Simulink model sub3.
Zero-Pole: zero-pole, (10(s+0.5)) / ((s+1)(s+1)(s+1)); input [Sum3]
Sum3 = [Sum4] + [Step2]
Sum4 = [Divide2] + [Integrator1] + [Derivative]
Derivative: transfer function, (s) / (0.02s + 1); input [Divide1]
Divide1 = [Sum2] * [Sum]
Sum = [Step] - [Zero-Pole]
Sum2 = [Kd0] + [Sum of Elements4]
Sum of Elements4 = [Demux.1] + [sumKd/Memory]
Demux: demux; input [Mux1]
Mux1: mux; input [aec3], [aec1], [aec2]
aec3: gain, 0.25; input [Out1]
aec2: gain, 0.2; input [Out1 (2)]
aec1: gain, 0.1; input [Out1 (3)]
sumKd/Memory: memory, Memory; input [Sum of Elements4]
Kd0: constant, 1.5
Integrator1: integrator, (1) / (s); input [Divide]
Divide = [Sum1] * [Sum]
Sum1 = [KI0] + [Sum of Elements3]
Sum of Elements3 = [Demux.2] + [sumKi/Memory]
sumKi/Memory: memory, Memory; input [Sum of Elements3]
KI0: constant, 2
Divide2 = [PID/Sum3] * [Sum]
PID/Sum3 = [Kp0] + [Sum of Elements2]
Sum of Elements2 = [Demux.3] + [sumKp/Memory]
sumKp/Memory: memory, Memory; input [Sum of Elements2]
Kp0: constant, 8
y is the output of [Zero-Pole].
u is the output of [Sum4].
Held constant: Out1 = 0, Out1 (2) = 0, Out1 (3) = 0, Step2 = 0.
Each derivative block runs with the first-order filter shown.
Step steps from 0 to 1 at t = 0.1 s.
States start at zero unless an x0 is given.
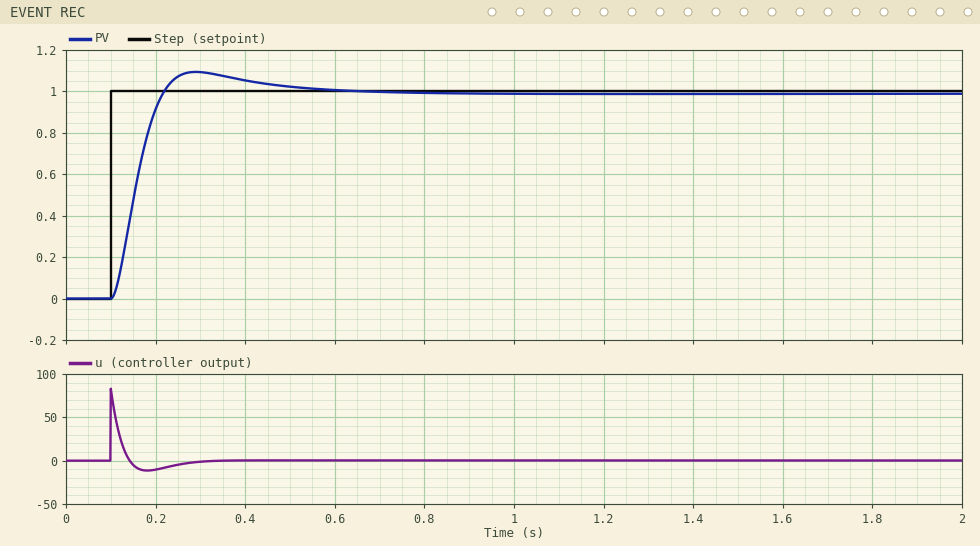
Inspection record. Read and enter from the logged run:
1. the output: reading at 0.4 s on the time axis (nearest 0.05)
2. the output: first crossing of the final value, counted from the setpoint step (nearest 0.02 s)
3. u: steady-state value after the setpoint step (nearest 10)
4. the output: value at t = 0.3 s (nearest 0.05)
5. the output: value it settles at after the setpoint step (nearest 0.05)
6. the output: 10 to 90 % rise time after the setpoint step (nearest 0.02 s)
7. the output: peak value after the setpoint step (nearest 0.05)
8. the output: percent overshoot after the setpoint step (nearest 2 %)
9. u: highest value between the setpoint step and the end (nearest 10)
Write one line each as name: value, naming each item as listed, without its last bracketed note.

the output: reading at 0.4 s on the time axis: 1.05
the output: first crossing of the final value, counted from the setpoint step: 0.12 s
u: steady-state value after the setpoint step: 0
the output: value at t = 0.3 s: 1.10
the output: value it settles at after the setpoint step: 1.00
the output: 10 to 90 % rise time after the setpoint step: 0.08 s
the output: peak value after the setpoint step: 1.10
the output: percent overshoot after the setpoint step: 10 %
u: highest value between the setpoint step and the end: 80
